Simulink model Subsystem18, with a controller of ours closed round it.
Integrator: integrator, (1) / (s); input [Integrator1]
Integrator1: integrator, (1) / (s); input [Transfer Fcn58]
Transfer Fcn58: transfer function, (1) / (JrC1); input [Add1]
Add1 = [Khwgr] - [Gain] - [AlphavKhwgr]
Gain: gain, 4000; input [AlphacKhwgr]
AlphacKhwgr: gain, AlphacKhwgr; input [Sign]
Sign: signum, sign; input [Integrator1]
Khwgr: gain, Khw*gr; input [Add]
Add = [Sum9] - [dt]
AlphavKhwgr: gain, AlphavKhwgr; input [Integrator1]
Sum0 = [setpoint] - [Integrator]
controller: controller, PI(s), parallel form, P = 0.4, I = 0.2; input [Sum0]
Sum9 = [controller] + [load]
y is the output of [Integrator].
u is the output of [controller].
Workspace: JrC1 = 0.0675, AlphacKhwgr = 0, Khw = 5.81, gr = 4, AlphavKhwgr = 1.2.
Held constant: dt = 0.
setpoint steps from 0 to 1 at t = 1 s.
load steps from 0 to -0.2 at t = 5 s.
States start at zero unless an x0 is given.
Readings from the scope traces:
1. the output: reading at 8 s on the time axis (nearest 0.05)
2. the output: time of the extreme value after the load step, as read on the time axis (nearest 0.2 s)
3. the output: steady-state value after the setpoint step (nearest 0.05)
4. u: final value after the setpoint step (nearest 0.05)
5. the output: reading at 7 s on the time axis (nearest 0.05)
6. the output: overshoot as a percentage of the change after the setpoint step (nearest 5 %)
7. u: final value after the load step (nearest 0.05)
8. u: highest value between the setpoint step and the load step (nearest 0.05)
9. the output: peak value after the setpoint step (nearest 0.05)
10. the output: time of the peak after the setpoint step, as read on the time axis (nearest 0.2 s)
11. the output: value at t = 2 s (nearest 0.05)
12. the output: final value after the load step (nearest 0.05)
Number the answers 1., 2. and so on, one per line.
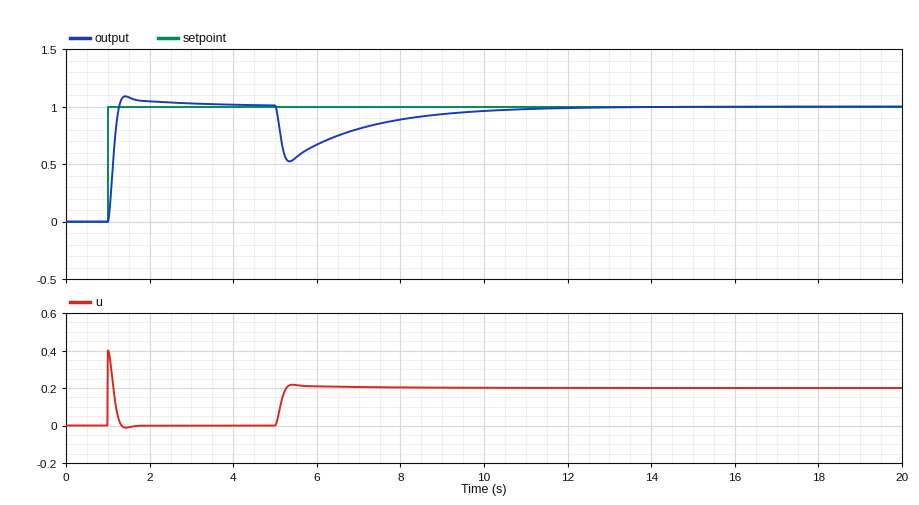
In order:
1. 0.90
2. 5.4 s
3. 1.00
4. 0.00
5. 0.80
6. 10 %
7. 0.20
8. 0.40
9. 1.10
10. 1.4 s
11. 1.05
12. 1.00
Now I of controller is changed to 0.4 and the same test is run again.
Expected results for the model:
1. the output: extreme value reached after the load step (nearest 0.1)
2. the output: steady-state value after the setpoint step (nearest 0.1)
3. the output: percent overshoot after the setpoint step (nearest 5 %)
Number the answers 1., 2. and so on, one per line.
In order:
1. 0.5
2. 1.0
3. 15 %
